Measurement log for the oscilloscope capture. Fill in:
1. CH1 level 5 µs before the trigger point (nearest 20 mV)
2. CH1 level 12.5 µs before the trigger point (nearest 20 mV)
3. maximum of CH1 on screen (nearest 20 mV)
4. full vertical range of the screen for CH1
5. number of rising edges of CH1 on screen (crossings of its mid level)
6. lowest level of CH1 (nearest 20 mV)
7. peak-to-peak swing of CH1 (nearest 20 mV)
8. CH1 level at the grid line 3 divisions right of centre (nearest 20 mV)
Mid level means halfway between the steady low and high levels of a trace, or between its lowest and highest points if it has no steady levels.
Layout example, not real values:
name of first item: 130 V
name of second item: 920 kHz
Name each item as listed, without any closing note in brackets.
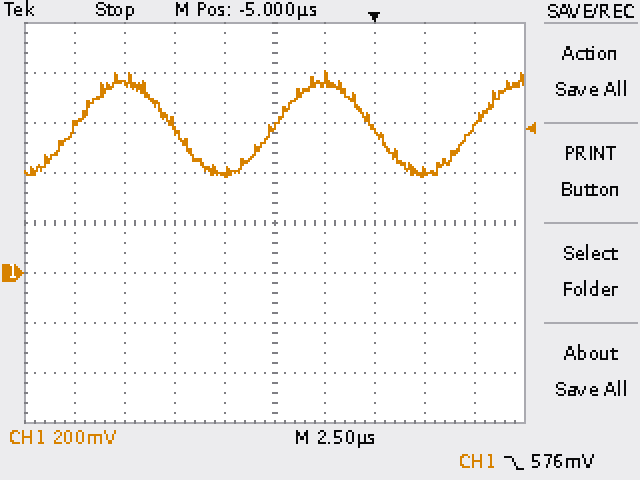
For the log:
CH1 level 5 µs before the trigger point: 580 mV
CH1 level 12.5 µs before the trigger point: 760 mV
maximum of CH1 on screen: 800 mV
full vertical range of the screen for CH1: 1.6 V
number of rising edges of CH1 on screen: 3
lowest level of CH1: 380 mV
peak-to-peak swing of CH1: 420 mV
CH1 level at the grid line 3 divisions right of centre: 400 mV
